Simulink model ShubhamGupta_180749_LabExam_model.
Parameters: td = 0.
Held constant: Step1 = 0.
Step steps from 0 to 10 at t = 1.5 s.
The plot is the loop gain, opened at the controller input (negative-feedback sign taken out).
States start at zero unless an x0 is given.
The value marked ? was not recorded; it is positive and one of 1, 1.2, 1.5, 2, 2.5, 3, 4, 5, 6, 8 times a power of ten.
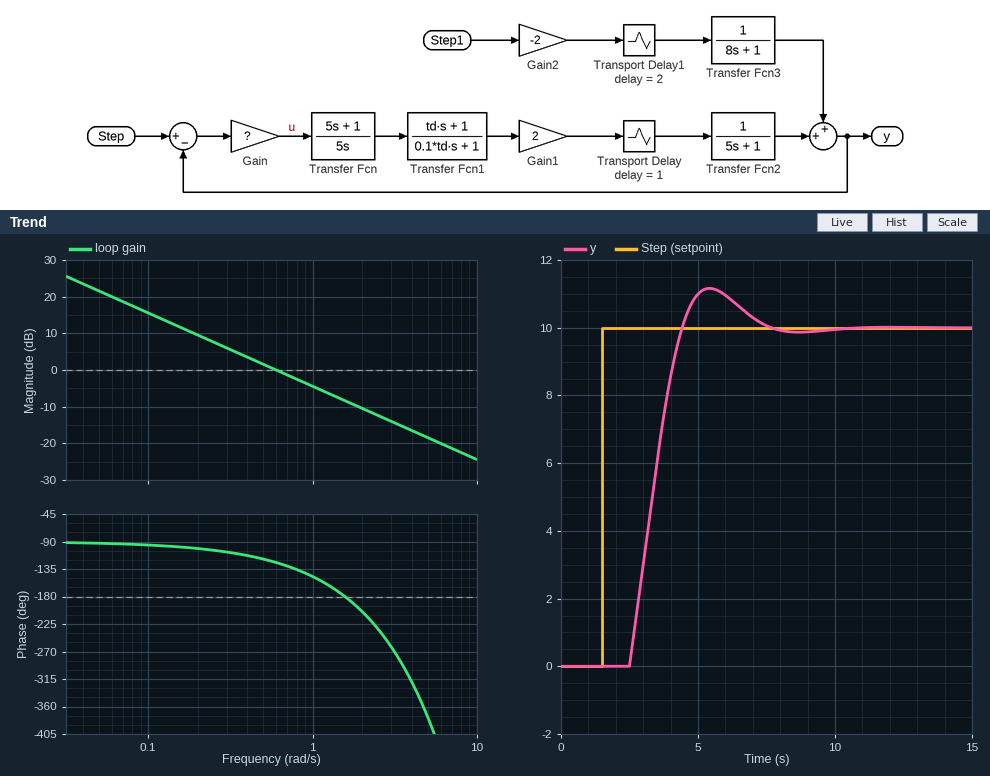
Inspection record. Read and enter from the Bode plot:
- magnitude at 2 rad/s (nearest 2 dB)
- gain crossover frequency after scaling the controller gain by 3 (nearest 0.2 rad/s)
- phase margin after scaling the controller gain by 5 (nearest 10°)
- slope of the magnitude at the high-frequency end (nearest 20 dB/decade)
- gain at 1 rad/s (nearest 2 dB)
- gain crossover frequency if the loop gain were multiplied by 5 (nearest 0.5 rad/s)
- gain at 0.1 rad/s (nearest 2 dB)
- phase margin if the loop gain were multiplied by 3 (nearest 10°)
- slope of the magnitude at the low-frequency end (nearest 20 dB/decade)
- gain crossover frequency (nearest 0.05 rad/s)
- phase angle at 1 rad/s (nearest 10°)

-10 dB
1.8 rad/s
-80°
-20 dB/decade
-4 dB
3.0 rad/s
16 dB
-10°
-20 dB/decade
0.60 rad/s
-150°
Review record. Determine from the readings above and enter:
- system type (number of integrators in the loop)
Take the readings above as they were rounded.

1
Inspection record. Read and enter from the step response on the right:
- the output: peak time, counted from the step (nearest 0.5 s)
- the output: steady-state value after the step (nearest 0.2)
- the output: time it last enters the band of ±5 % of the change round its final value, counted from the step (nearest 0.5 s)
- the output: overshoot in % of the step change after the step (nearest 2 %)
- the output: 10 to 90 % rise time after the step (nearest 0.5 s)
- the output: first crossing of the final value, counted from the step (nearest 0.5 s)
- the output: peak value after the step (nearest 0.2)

4.0 s
10.0
5.0 s
12 %
1.5 s
3.0 s
11.2
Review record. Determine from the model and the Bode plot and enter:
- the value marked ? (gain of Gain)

1.5
